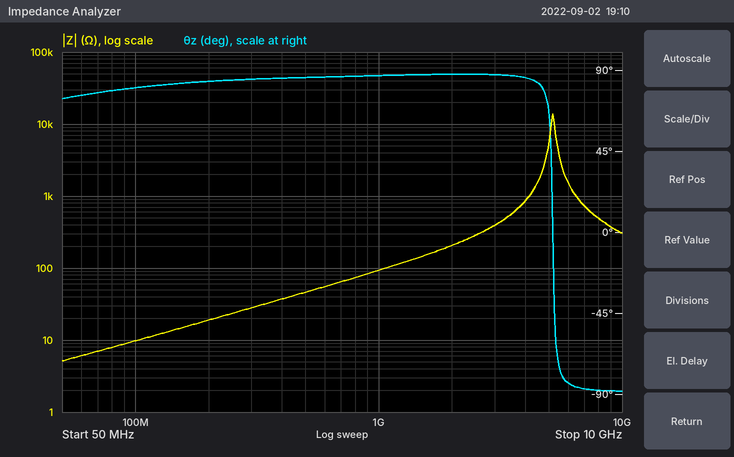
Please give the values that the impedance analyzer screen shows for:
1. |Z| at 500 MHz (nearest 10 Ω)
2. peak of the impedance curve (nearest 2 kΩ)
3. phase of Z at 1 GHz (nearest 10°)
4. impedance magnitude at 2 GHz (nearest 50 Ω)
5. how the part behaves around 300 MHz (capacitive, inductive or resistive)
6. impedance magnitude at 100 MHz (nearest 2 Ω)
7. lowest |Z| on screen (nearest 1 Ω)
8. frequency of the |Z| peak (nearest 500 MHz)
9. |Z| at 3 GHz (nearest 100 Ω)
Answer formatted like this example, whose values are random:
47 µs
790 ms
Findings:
50 Ω
14 kΩ
90°
200 Ω
inductive
10 Ω
5 Ω
5.0 GHz
400 Ω
